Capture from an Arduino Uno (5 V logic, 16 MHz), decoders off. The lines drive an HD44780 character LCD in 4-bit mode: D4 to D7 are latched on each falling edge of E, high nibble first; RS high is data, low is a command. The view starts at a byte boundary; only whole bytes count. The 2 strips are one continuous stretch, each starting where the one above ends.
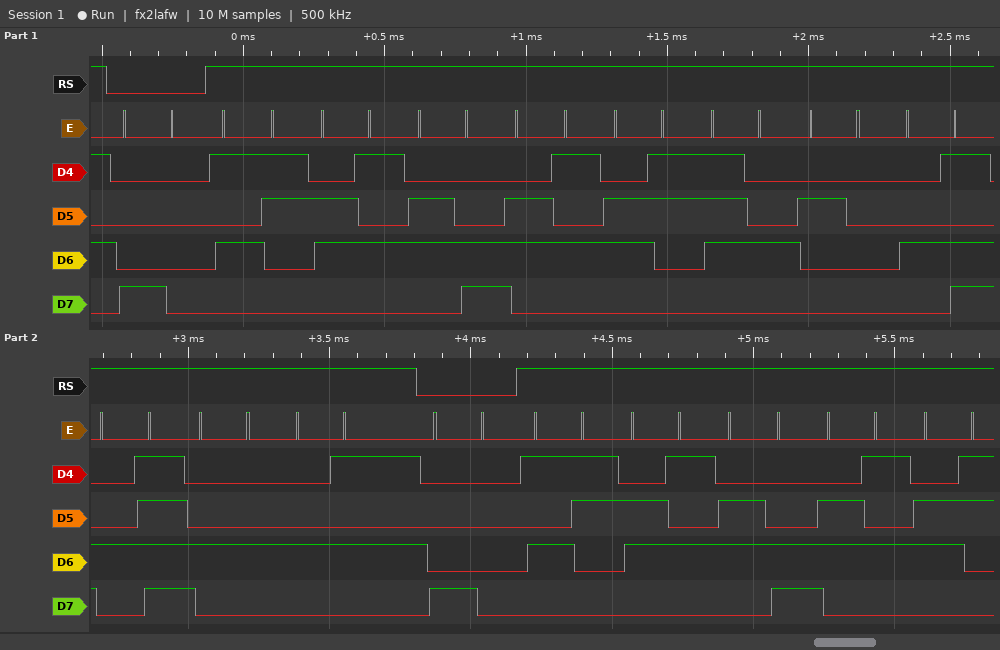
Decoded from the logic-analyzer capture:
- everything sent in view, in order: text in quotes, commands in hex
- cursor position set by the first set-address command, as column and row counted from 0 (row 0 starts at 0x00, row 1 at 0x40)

0x80 "Select MODE" 0x80 "Selec"
column 0, row 0
